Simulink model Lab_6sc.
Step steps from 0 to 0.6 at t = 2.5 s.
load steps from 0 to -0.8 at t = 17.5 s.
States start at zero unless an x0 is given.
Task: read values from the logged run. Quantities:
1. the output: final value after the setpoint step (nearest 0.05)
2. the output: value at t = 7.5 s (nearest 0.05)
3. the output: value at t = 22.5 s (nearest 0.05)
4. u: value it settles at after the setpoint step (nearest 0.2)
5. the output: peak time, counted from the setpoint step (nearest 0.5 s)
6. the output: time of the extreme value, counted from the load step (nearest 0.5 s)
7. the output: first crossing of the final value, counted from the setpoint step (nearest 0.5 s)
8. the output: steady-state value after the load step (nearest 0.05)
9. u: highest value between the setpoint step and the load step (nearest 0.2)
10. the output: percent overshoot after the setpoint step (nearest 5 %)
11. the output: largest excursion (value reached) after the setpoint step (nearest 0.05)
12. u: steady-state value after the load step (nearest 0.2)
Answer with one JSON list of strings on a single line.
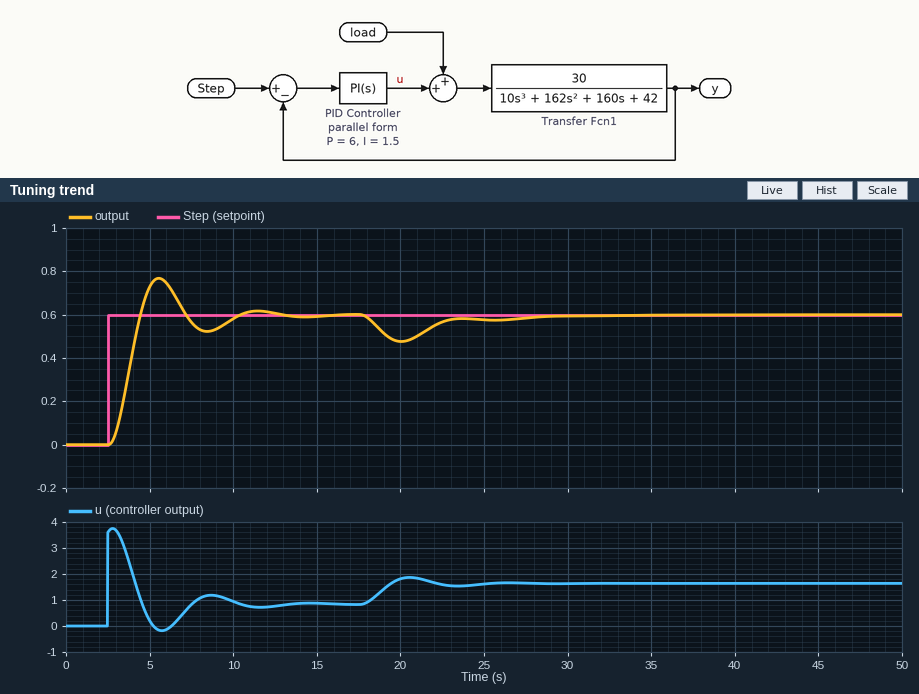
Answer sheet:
["0.60", "0.55", "0.55", "0.8", "3.0 s", "2.5 s", "2.0 s", "0.60", "3.8", "30 %", "0.75", "1.6"]
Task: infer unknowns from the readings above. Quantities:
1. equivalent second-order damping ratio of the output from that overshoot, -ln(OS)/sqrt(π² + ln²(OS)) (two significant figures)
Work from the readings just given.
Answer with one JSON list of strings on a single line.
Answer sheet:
["0.36"]
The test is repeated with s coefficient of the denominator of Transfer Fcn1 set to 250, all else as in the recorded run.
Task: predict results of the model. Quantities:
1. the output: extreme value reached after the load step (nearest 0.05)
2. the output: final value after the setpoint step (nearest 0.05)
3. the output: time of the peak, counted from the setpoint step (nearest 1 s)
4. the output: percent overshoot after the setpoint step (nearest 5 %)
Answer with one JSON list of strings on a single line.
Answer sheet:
["0.50", "0.60", "4 s", "15 %"]
